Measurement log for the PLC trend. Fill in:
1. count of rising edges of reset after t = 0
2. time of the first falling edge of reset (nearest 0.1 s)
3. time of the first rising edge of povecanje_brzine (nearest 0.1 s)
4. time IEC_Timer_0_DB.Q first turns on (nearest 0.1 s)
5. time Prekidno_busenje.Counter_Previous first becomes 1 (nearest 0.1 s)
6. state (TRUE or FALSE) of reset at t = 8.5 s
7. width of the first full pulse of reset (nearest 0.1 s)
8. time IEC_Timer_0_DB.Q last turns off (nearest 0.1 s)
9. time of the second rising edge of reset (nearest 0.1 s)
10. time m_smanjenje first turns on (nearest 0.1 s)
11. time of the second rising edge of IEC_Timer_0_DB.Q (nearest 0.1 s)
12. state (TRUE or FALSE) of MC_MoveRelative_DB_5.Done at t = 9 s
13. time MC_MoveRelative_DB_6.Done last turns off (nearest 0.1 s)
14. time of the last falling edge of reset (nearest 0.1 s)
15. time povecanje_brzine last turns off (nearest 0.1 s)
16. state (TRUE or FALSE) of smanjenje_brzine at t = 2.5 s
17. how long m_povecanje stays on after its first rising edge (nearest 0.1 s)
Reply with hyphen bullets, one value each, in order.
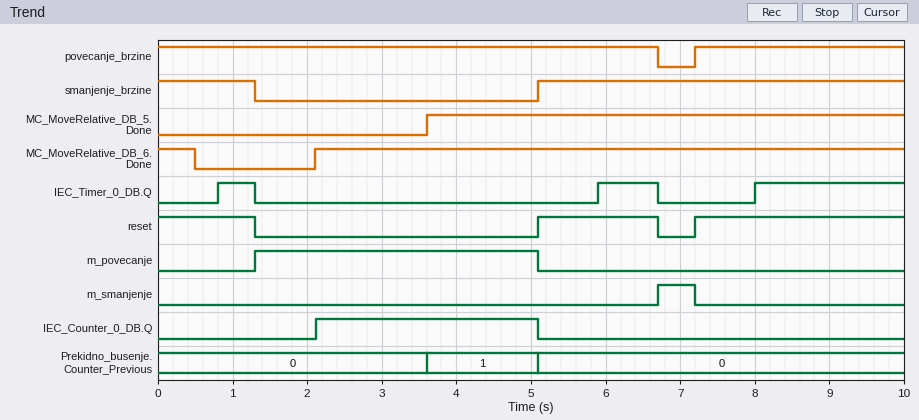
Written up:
- 2
- 1.3 s
- 7.2 s
- 0.8 s
- 3.6 s
- TRUE
- 1.6 s
- 6.7 s
- 7.2 s
- 6.7 s
- 5.9 s
- TRUE
- 0.5 s
- 6.7 s
- 6.7 s
- FALSE
- 3.8 s
